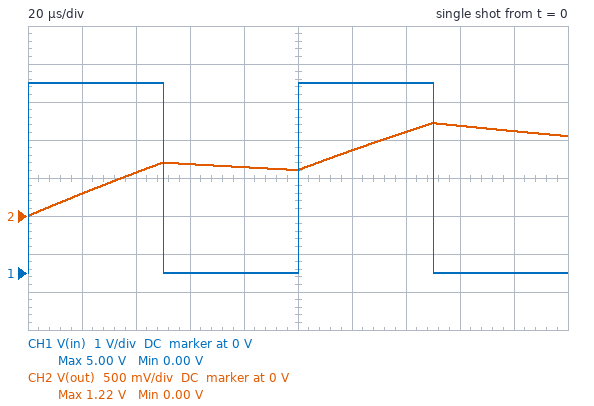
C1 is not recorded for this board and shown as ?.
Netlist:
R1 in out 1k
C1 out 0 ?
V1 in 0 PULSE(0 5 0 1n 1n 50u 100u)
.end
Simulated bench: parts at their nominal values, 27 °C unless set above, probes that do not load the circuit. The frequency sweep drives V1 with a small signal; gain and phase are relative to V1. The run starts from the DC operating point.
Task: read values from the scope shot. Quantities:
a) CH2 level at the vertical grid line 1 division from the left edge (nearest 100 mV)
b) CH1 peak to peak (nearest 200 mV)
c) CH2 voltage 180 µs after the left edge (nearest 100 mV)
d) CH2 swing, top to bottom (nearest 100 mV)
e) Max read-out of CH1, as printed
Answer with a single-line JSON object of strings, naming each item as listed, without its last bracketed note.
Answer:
{"CH2 level at the vertical grid line 1 division from the left edge": "300 mV", "CH1 peak to peak": "5.0 V", "CH2 voltage 180 µs after the left edge": "1.1 V", "CH2 swing, top to bottom": "1.2 V", "Max read-out of CH1, as printed": "5.00 V"}
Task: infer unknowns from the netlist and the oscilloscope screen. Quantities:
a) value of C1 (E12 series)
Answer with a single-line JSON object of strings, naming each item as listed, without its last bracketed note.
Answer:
{"value of C1": "330 nF"}
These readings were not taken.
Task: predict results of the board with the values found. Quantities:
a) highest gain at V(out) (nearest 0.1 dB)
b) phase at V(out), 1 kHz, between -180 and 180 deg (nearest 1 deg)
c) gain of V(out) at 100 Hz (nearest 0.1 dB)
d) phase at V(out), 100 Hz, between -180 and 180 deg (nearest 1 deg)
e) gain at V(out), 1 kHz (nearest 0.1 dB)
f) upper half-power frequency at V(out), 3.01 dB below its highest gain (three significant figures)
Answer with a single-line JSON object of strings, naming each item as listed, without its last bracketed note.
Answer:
{"highest gain at V(out)": "0 dB", "phase at V(out), 1 kHz, between -180 and 180 deg": "-64 deg", "gain of V(out) at 100 Hz": "-0.2 dB", "phase at V(out), 100 Hz, between -180 and 180 deg": "-12 deg", "gain at V(out), 1 kHz": "-7.2 dB", "upper half-power frequency at V(out), 3.01 dB below its highest gain": "482 Hz"}
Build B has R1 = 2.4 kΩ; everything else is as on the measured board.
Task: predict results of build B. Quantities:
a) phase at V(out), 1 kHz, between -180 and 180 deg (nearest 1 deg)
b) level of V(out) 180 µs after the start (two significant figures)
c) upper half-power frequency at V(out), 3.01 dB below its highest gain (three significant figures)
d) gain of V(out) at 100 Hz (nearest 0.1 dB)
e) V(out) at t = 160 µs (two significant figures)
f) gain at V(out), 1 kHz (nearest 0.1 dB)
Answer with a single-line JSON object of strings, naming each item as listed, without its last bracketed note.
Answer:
{"phase at V(out), 1 kHz, between -180 and 180 deg": "-79 deg", "level of V(out) 180 µs after the start": "550 mV", "upper half-power frequency at V(out), 3.01 dB below its highest gain": "201 Hz", "gain of V(out) at 100 Hz": "-1.0 dB", "V(out) at t = 160 µs": "570 mV", "gain at V(out), 1 kHz": "-14.1 dB"}
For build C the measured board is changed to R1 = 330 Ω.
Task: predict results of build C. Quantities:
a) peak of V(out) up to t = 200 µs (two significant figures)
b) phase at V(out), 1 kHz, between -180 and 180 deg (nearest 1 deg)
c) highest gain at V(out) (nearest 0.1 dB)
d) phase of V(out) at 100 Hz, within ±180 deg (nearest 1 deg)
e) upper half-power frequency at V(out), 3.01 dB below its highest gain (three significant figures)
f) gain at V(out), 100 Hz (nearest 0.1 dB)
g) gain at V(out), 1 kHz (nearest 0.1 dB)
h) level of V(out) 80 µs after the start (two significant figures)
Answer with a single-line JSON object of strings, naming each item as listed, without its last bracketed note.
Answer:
{"peak of V(out) up to t = 200 µs": "2.6 V", "phase at V(out), 1 kHz, between -180 and 180 deg": "-34 deg", "highest gain at V(out)": "0 dB", "phase of V(out) at 100 Hz, within ±180 deg": "-4 deg", "upper half-power frequency at V(out), 3.01 dB below its highest gain": "1.46 kHz", "gain at V(out), 100 Hz": "0 dB", "gain at V(out), 1 kHz": "-1.7 dB", "level of V(out) 80 µs after the start": "1.4 V"}
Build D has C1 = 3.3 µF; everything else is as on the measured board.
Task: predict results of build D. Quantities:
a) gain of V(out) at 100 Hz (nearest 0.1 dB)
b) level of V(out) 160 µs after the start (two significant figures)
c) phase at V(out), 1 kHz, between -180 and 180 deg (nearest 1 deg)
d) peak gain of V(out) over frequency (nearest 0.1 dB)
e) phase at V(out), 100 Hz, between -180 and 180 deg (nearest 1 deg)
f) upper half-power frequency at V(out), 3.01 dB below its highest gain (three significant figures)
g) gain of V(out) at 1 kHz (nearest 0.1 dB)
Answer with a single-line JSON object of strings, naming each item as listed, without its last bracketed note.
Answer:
{"gain of V(out) at 100 Hz": "-7.2 dB", "level of V(out) 160 µs after the start": "150 mV", "phase at V(out), 1 kHz, between -180 and 180 deg": "-87 deg", "peak gain of V(out) over frequency": "0 dB", "phase at V(out), 100 Hz, between -180 and 180 deg": "-64 deg", "upper half-power frequency at V(out), 3.01 dB below its highest gain": "48.2 Hz", "gain of V(out) at 1 kHz": "-26.3 dB"}
